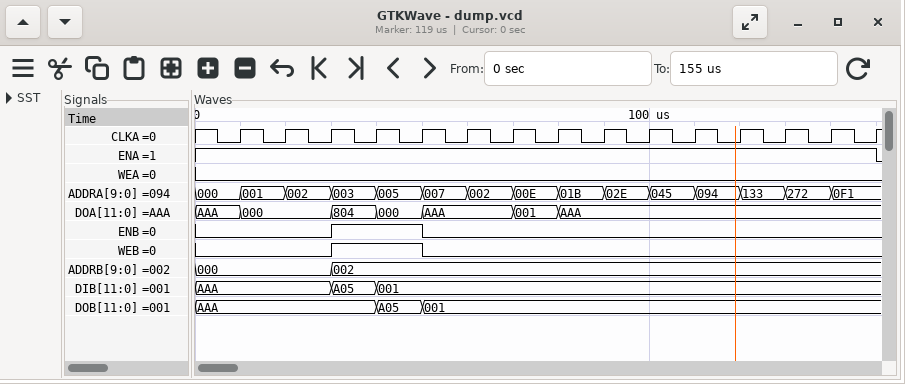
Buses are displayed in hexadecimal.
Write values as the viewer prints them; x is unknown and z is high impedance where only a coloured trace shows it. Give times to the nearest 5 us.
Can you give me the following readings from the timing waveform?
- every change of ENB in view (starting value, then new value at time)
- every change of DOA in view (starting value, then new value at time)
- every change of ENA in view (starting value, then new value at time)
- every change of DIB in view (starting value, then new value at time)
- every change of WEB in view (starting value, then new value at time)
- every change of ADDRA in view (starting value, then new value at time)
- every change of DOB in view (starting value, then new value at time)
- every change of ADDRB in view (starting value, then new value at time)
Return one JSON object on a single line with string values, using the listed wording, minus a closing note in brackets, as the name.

{"every change of ENB in view": "0, 1 at 30 us, 0 at 50 us", "every change of DOA in view": "AAA, 000 at 10 us, 804 at 30 us, 000 at 40 us, AAA at 50 us, 001 at 70 us, AAA at 80 us", "every change of ENA in view": "1, 0 at 150 us", "every change of DIB in view": "AAA, A05 at 30 us, 001 at 40 us", "every change of WEB in view": "0, 1 at 30 us, 0 at 50 us", "every change of ADDRA in view": "000, 001 at 10 us, 002 at 20 us, 003 at 30 us, 005 at 40 us, 007 at 50 us, 002 at 60 us, 00E at 70 us, 01B at 80 us, 02E at 90 us, 045 at 100 us, 094 at 110 us, 133 at 120 us, 272 at 130 us, 0F1 at 140 us", "every change of DOB in view": "AAA, A05 at 40 us, 001 at 50 us", "every change of ADDRB in view": "000, 002 at 30 us"}
